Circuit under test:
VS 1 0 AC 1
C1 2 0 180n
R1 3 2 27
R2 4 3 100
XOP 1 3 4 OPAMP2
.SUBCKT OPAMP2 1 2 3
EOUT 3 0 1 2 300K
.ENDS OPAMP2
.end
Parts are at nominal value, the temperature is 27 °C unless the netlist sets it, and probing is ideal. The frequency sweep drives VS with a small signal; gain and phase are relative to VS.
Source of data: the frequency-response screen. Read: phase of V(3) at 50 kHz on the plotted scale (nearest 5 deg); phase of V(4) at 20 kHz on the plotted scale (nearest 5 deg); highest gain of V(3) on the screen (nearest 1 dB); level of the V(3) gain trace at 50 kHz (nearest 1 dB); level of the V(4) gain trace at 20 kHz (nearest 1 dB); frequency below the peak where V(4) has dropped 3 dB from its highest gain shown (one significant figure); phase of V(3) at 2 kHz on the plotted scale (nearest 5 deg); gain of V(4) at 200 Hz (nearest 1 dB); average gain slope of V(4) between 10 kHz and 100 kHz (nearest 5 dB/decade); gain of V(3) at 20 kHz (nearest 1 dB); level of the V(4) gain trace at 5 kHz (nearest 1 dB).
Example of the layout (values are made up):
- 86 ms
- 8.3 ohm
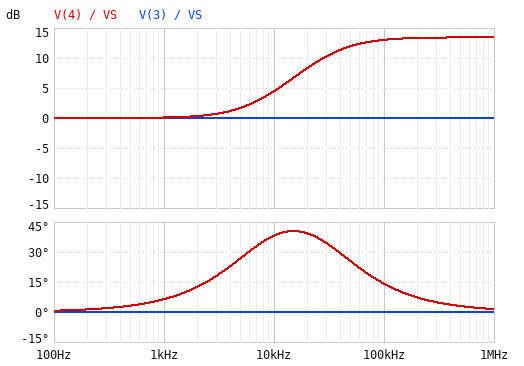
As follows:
- 0 deg
- 40 deg
- 0 dB
- 0 dB
- 8 dB
- 30 kHz
- 0 deg
- 0 dB
- 10 dB/decade
- 0 dB
- 2 dB
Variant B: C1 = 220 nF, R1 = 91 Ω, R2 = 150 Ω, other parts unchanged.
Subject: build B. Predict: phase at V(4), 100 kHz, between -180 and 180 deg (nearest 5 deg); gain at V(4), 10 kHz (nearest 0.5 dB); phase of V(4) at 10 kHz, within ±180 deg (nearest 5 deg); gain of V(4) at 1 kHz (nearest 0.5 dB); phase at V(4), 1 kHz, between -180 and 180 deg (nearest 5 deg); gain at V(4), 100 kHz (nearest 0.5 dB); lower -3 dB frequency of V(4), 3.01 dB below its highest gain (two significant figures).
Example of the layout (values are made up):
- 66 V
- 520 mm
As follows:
- 5 deg
- 6.5 dB
- 20 deg
- 0.5 dB
- 10 deg
- 8.5 dB
- 6.7 kHz
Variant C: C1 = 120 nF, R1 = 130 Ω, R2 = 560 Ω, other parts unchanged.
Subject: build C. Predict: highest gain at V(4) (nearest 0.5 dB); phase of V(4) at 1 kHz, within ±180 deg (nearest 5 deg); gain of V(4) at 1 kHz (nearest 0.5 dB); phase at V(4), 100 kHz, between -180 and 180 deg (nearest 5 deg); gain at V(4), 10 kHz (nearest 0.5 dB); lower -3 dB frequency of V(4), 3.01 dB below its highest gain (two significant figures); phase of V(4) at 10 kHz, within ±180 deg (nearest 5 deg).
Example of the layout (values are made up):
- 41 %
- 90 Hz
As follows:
- 14.5 dB
- 20 deg
- 1.0 dB
- 5 deg
- 11.5 dB
- 9.8 kHz
- 35 deg
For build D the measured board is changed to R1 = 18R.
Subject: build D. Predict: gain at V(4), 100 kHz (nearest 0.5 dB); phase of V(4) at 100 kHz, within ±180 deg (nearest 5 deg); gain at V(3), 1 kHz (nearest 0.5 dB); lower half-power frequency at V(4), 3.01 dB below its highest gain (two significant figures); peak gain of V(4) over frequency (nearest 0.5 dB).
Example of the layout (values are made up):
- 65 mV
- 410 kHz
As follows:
- 15.5 dB
- 20 deg
- 0 dB
- 48 kHz
- 16.5 dB
